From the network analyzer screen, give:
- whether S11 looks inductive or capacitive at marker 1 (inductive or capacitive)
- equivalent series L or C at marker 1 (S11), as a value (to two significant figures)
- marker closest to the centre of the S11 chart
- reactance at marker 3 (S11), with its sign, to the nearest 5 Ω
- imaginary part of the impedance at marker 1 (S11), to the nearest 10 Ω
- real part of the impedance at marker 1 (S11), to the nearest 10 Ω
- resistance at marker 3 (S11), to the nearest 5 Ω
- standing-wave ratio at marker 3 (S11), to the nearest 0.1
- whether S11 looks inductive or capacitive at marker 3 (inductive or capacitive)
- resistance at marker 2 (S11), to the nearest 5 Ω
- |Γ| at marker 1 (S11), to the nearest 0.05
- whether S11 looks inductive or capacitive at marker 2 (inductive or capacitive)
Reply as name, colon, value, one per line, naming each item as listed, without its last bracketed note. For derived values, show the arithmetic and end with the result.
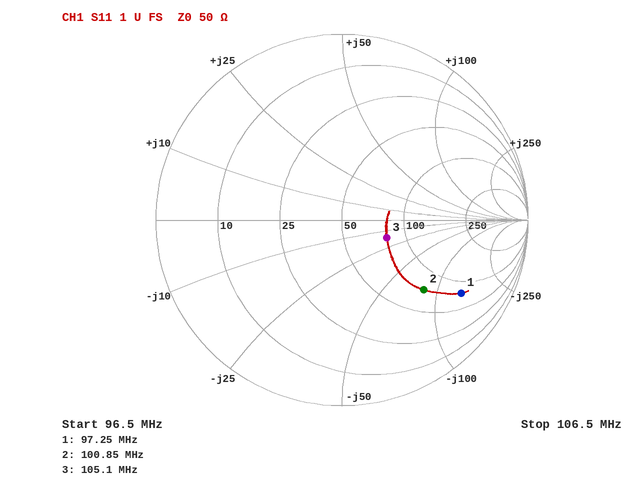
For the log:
whether S11 looks inductive or capacitive at marker 1: capacitive
equivalent series L or C at marker 1 (S11), as a value: C = 1/(2π × 97.25 MHz × 140 Ω) ≈ 12 pF
marker closest to the centre of the S11 chart: marker 3
reactance at marker 3 (S11), with its sign, to the nearest 5 Ω: -15 Ω
imaginary part of the impedance at marker 1 (S11), to the nearest 10 Ω: -140 Ω
real part of the impedance at marker 1 (S11), to the nearest 10 Ω: 80 Ω
resistance at marker 3 (S11), to the nearest 5 Ω: 80 Ω
standing-wave ratio at marker 3 (S11), to the nearest 0.1: 1.7
whether S11 looks inductive or capacitive at marker 3: capacitive
resistance at marker 2 (S11), to the nearest 5 Ω: 75 Ω
|Γ| at marker 1 (S11), to the nearest 0.05: 0.75
whether S11 looks inductive or capacitive at marker 2: capacitive
